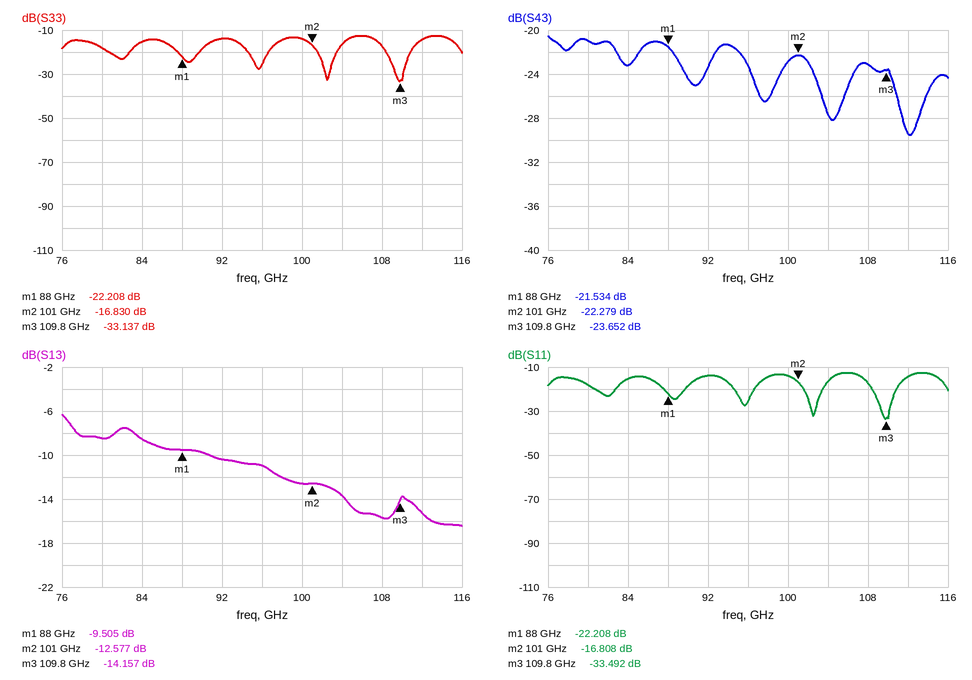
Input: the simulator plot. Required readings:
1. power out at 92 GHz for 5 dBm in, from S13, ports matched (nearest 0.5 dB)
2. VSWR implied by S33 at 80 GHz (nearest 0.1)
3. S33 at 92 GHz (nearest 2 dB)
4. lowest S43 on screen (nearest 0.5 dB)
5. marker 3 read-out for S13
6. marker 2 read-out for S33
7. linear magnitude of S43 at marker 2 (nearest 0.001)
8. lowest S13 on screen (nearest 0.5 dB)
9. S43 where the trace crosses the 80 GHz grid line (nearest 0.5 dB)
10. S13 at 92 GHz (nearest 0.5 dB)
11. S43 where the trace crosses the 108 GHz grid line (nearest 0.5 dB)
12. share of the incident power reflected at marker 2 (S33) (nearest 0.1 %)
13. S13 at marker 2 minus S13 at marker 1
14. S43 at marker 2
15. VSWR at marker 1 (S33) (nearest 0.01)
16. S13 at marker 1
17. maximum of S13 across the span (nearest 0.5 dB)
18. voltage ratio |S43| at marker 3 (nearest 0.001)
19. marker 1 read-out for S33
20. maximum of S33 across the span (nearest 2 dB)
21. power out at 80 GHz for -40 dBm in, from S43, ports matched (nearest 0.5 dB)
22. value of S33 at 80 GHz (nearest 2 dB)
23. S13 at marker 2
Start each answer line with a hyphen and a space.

- -5.5 dBm
- 1.3
- -14 dB
- -29.5 dB
- -14.157 dB
- -16.830 dB
- 0.077
- -16.5 dB
- -21.0 dB
- -10.5 dB
- -23.0 dB
- 2.1 %
- -3.072 dB
- -22.279 dB
- 1.17
- -9.505 dB
- -6.5 dB
- 0.066
- -22.208 dB
- -12 dB
- -61.0 dBm
- -18 dB
- -12.577 dB
